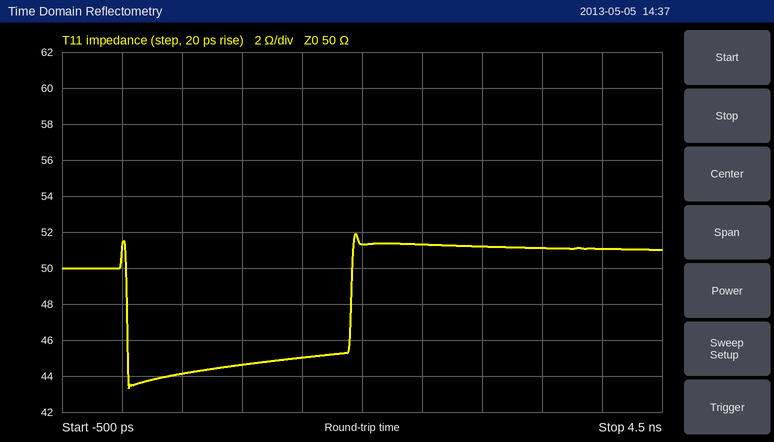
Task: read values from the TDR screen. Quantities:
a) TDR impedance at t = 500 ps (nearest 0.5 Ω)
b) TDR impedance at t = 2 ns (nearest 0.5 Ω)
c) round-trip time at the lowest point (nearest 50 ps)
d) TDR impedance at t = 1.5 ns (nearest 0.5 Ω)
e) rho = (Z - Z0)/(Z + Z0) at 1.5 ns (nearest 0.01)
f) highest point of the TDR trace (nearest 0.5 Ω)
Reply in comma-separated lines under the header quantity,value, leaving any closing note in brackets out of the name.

quantity,value
TDR impedance at t = 500 ps,44.0 Ω
TDR impedance at t = 2 ns,51.5 Ω
round-trip time at the lowest point,50 ps
TDR impedance at t = 1.5 ns,45.0 Ω
rho = (Z - Z0)/(Z + Z0) at 1.5 ns,-0.05
highest point of the TDR trace,52.0 Ω
